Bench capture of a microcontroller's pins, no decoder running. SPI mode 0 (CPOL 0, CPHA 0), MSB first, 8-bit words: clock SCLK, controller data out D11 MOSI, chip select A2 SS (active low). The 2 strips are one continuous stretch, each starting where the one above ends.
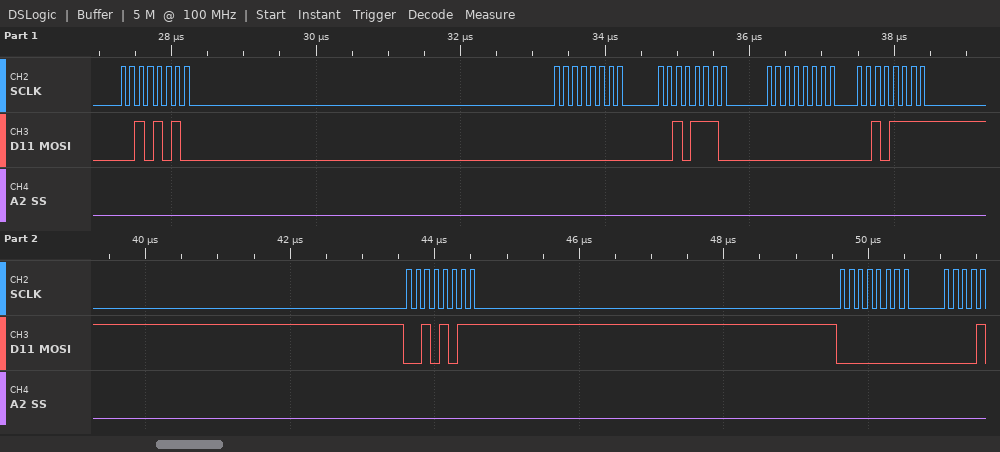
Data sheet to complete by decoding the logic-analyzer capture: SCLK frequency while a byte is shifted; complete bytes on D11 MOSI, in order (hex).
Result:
8 MHz
2A 00 2E 00 2F 2B 00
